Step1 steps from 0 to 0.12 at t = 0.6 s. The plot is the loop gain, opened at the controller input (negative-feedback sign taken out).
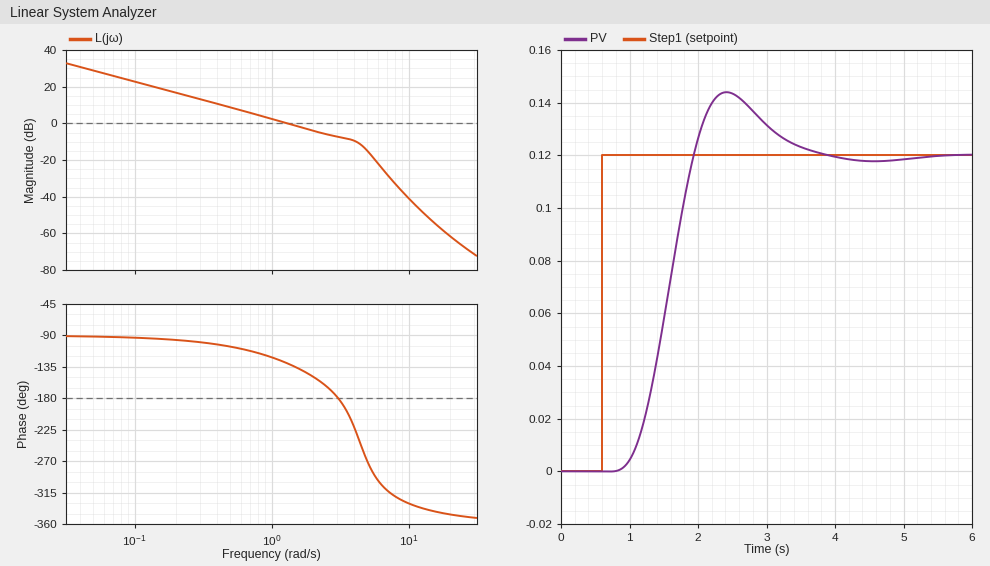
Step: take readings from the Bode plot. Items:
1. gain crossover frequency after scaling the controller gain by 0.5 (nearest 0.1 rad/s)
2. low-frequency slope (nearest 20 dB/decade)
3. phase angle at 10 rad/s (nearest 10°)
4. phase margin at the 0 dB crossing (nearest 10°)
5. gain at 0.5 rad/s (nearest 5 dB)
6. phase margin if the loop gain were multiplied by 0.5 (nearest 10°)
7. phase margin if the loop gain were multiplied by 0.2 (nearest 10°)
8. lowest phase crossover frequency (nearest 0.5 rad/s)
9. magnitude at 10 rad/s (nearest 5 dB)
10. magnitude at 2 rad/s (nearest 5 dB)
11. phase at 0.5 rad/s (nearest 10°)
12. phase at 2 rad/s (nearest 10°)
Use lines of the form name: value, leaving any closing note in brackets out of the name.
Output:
gain crossover frequency after scaling the controller gain by 0.5: 0.7 rad/s
low-frequency slope: -20 dB/decade
phase angle at 10 rad/s: -330°
phase margin at the 0 dB crossing: 50°
gain at 0.5 rad/s: 10 dB
phase margin if the loop gain were multiplied by 0.5: 70°
phase margin if the loop gain were multiplied by 0.2: 80°
lowest phase crossover frequency: 3.0 rad/s
magnitude at 10 rad/s: -40 dB
magnitude at 2 rad/s: -5 dB
phase at 0.5 rad/s: -110°
phase at 2 rad/s: -150°
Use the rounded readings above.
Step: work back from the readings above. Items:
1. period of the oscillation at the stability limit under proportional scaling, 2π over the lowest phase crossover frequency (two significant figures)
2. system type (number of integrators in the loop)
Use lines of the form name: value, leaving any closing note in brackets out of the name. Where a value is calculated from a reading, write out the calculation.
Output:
period of the oscillation at the stability limit under proportional scaling, 2π over the lowest phase crossover frequency: 2π / 3 = 2.1 s
system type: 1
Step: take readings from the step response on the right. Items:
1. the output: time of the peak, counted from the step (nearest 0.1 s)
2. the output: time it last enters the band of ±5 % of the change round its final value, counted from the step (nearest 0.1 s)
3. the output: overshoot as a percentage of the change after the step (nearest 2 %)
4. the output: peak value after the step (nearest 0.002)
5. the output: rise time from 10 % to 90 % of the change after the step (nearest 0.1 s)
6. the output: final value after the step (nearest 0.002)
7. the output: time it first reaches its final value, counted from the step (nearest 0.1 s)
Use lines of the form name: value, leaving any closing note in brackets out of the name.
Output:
the output: time of the peak, counted from the step: 1.8 s
the output: time it last enters the band of ±5 % of the change round its final value, counted from the step: 2.7 s
the output: overshoot as a percentage of the change after the step: 20 %
the output: peak value after the step: 0.144
the output: rise time from 10 % to 90 % of the change after the step: 0.7 s
the output: final value after the step: 0.120
the output: time it first reaches its final value, counted from the step: 1.3 s
